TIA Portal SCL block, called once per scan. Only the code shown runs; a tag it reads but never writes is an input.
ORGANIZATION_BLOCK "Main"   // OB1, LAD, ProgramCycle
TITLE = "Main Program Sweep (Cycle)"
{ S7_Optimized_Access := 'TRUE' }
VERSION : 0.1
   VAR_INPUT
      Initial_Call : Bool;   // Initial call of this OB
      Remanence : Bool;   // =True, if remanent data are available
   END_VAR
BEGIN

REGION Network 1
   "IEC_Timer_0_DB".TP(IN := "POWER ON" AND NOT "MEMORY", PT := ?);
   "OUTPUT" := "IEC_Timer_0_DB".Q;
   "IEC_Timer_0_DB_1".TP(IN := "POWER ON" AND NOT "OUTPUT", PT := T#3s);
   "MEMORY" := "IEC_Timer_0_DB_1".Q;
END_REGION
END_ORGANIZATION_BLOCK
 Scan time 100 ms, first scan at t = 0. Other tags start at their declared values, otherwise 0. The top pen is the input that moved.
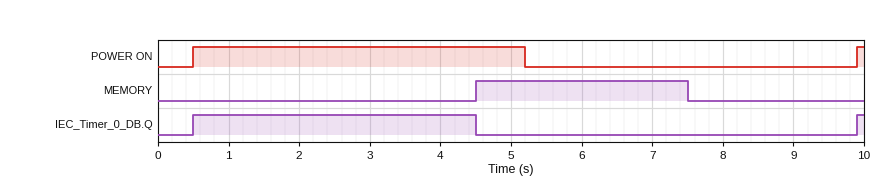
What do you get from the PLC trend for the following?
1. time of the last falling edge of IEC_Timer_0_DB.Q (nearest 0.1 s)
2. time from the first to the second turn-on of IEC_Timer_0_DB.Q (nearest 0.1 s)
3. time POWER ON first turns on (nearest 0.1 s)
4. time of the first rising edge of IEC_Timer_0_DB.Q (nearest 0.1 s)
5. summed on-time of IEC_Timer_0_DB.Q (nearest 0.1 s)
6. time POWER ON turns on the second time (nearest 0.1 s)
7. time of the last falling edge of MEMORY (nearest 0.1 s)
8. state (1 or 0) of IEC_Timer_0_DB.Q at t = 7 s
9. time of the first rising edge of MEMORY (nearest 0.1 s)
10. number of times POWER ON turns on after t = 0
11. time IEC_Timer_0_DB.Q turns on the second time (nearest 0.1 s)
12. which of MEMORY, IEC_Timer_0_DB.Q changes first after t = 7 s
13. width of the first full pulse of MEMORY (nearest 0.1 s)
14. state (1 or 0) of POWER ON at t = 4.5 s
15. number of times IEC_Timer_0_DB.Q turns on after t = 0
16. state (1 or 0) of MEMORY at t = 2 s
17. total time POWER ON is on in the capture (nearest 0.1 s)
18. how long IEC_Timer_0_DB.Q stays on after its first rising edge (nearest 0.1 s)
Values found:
4.5 s
9.4 s
0.5 s
0.5 s
4.1 s
9.9 s
7.5 s
0
4.5 s
2
9.9 s
MEMORY
3.0 s
1
2
0
4.8 s
4.0 s
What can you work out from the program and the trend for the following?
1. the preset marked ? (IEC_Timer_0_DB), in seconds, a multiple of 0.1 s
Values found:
4.0 s
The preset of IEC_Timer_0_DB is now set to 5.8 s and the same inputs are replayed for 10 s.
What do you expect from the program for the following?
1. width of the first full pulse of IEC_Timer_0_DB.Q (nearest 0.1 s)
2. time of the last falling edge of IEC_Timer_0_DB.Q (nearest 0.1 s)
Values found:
5.8 s
6.3 s
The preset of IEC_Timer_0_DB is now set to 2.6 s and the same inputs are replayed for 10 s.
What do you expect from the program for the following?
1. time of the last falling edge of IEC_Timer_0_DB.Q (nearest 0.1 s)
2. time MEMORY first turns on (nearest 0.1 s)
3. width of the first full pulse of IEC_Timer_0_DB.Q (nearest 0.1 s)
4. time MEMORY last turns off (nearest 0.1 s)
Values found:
3.1 s
3.1 s
2.6 s
6.1 s
